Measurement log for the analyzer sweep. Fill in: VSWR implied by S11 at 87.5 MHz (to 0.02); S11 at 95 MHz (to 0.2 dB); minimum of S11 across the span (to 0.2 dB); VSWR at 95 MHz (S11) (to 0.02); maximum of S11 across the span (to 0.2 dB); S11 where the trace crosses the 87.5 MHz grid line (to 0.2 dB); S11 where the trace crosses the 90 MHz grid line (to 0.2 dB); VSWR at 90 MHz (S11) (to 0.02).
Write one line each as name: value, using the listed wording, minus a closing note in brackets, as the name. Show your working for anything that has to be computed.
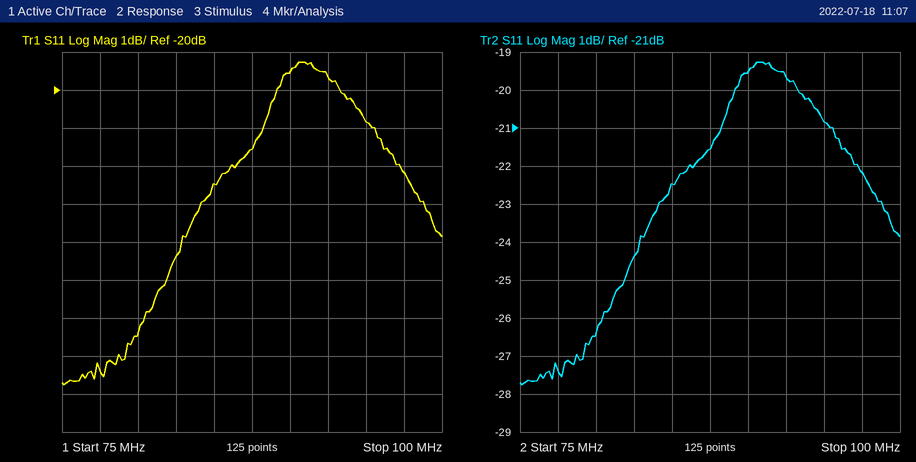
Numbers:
VSWR implied by S11 at 87.5 MHz: |Γ| = 10^(-21.6/20) = 0.0832; VSWR = (1 + 0.0832)/(1 − 0.0832) ≈ 1.18
S11 at 95 MHz: -20.8 dB
minimum of S11 across the span: -27.8 dB
VSWR at 95 MHz (S11): |Γ| = 10^(-20.8/20) = 0.0912; VSWR = (1 + 0.0912)/(1 − 0.0912) ≈ 1.20
maximum of S11 across the span: -19.2 dB
S11 where the trace crosses the 87.5 MHz grid line: -21.6 dB
S11 where the trace crosses the 90 MHz grid line: -19.6 dB
VSWR at 90 MHz (S11): |Γ| = 10^(-19.6/20) = 0.1047; VSWR = (1 + 0.1047)/(1 − 0.1047) ≈ 1.23, so 1.24 to the nearest 0.02
